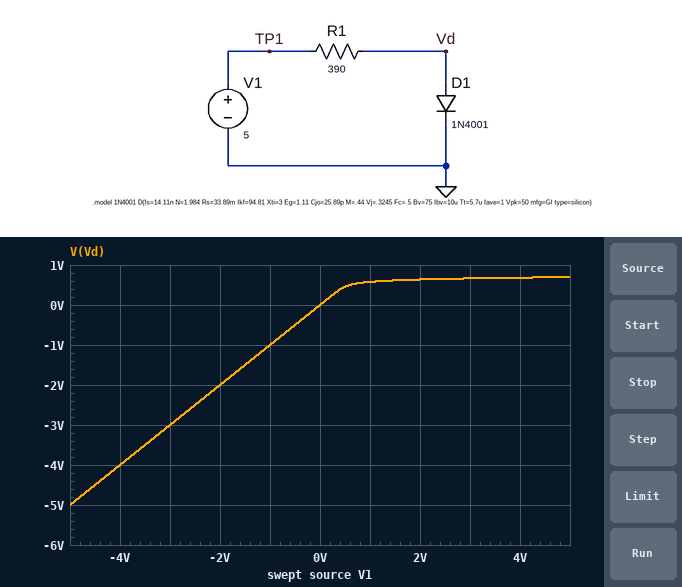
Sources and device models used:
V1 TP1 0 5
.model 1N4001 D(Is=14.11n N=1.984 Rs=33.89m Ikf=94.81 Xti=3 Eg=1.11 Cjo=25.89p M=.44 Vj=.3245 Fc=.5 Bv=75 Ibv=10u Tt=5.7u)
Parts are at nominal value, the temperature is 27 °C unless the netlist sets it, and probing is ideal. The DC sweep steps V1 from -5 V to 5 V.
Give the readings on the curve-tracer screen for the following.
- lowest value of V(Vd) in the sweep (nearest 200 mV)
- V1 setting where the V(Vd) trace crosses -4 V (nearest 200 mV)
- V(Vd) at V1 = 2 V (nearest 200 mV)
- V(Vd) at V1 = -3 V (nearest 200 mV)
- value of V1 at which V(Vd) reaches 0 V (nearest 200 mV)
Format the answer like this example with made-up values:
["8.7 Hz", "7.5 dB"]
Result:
["-5.0 V", "-4.0 V", "600 mV", "-3.0 V", "0 V"]
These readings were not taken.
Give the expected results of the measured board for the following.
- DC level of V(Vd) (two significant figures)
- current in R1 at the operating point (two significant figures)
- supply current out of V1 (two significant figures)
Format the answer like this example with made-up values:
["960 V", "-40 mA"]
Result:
["700 mV", "11 mA", "11 mA"]
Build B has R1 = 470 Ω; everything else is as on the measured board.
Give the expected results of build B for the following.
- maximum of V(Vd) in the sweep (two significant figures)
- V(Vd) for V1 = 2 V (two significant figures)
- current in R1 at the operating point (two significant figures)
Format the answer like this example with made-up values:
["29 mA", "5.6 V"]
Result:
["690 mV", "630 mV", "9.2 mA"]
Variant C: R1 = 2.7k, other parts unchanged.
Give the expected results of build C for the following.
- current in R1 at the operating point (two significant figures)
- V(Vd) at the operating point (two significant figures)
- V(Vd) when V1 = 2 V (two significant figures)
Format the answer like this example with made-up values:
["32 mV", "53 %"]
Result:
["1.6 mA", "600 mV", "540 mV"]
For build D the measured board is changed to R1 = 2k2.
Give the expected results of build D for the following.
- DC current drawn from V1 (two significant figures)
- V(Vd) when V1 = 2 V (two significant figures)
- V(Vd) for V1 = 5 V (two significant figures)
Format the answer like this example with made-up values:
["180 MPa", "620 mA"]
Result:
["2.0 mA", "550 mV", "610 mV"]
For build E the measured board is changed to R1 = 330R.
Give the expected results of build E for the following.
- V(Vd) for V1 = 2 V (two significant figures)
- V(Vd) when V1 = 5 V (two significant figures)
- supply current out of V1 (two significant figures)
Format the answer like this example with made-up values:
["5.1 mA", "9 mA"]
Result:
["650 mV", "710 mV", "13 mA"]
